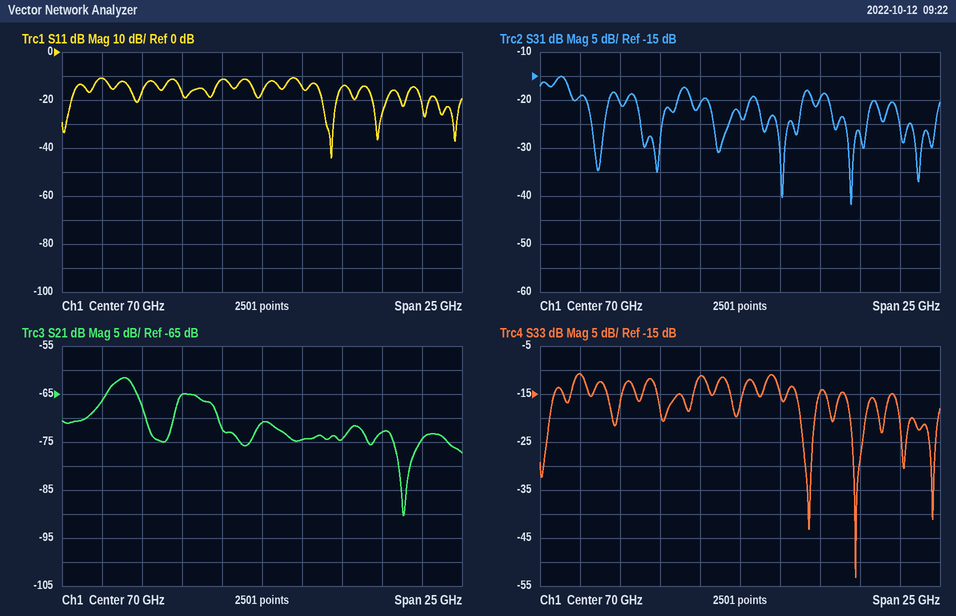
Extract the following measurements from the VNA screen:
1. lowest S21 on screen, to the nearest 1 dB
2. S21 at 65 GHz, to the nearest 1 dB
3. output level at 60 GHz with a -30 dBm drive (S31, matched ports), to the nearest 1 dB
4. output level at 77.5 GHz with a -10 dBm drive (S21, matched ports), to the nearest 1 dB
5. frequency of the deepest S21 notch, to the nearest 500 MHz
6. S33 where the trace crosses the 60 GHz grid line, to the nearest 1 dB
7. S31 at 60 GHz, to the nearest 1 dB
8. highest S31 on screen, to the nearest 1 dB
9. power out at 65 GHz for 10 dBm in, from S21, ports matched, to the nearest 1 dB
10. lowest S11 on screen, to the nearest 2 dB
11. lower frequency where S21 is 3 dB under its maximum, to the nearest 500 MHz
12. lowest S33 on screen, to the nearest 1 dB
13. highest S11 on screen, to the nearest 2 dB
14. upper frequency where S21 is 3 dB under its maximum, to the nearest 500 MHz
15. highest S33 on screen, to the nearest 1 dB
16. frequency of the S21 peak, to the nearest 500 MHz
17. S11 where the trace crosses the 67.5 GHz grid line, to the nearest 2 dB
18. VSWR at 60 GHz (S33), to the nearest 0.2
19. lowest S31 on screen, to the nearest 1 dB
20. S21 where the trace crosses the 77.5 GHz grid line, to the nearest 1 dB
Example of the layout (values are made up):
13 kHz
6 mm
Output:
-90 dB
-65 dB
-49 dBm
-83 dBm
79.0 GHz
-11 dB
-19 dB
-15 dB
-55 dBm
-44 dB
60.5 GHz
-53 dB
-10 dB
62.0 GHz
-11 dB
61.5 GHz
-12 dB
1.8
-42 dB
-73 dB
